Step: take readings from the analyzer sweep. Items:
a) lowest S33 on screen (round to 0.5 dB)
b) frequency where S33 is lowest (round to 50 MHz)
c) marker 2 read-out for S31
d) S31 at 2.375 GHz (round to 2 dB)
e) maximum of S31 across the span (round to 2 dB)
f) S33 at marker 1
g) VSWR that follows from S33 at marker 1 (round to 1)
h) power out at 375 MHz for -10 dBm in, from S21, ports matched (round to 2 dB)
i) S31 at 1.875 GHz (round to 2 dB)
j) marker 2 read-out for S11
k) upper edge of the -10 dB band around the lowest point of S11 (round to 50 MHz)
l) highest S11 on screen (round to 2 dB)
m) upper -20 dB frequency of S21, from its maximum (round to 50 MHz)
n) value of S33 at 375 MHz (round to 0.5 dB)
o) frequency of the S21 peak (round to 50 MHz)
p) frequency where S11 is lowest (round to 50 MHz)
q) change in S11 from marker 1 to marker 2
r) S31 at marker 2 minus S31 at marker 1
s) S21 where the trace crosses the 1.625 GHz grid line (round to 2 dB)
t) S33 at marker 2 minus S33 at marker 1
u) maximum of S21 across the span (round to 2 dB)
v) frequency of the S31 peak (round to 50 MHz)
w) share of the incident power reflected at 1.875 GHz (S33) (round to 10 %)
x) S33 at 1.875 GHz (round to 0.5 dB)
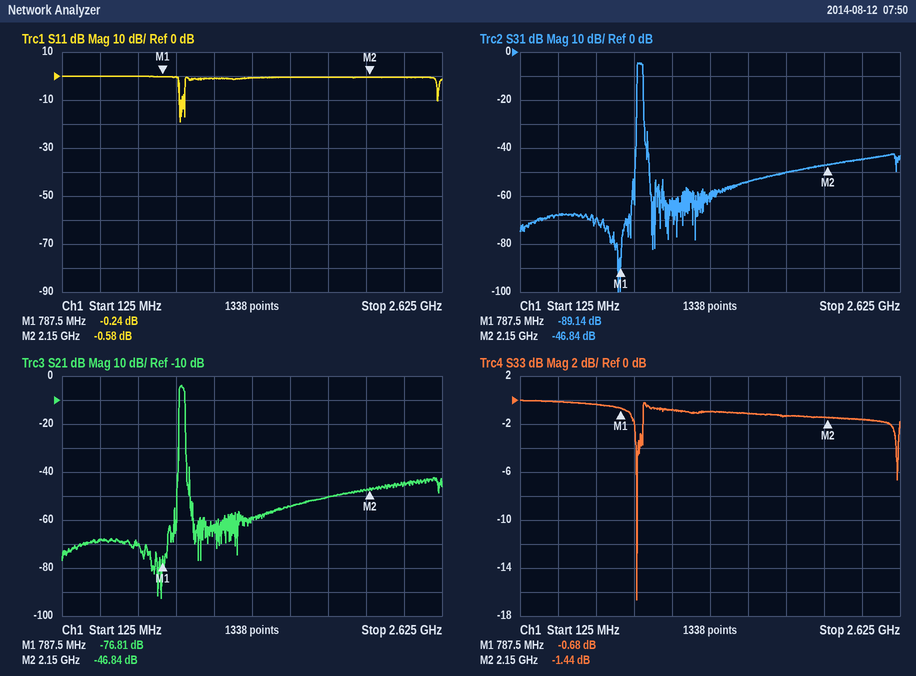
-16.5 dB
900 MHz
-46.84 dB
-44 dB
-4 dB
-0.68 dB
26
-78 dBm
-50 dB
-0.58 dB
900 MHz
0 dB
950 MHz
0.0 dB
900 MHz
900 MHz
-0.34 dB
42.30 dB
-54 dB
-0.76 dB
-4 dB
900 MHz
70 %
-1.5 dB
